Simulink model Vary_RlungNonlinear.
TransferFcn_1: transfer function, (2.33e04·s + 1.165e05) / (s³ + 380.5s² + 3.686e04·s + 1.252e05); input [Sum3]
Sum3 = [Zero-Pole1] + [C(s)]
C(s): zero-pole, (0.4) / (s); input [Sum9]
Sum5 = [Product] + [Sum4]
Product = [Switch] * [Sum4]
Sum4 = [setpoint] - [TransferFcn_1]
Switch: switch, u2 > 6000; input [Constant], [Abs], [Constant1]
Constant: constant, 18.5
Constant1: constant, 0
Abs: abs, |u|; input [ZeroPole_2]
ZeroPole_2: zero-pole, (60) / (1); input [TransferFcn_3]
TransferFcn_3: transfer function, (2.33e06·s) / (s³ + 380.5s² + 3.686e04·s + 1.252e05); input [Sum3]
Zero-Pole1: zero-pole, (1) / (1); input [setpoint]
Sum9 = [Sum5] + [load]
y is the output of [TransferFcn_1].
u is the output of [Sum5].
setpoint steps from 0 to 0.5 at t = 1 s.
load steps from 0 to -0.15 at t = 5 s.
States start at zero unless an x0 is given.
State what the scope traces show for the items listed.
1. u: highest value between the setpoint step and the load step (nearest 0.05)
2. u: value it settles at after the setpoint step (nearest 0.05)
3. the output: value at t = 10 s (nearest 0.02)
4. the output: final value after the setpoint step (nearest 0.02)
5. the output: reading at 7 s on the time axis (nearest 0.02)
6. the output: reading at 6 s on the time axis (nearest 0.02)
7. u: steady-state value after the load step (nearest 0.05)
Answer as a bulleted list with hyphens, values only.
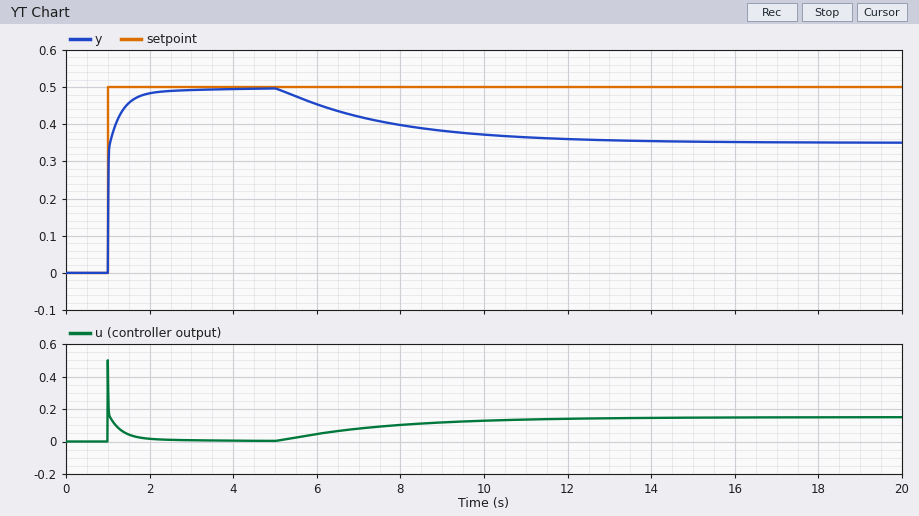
- 0.50
- 0.00
- 0.38
- 0.50
- 0.42
- 0.46
- 0.15
